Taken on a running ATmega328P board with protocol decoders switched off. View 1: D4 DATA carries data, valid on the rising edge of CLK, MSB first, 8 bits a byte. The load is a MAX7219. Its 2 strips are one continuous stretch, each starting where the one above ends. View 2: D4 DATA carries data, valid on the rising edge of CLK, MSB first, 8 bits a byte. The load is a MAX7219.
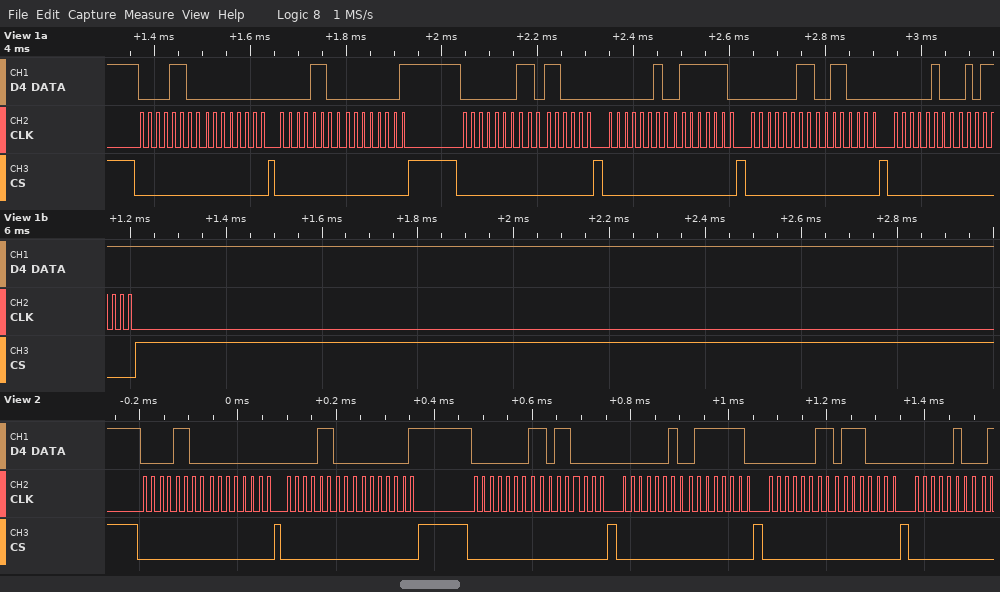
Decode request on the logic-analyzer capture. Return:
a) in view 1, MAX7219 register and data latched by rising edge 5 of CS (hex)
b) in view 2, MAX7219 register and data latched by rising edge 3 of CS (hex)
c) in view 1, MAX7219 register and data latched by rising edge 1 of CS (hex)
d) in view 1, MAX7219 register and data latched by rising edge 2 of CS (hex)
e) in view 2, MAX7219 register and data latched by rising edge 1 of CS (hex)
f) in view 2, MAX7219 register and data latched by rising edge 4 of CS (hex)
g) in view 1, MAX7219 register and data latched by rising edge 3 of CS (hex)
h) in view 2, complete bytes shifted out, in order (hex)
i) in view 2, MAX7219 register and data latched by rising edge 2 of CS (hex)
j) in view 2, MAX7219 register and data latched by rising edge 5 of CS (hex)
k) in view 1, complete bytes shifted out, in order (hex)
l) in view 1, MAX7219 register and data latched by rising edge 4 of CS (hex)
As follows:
register 0x3, data 0x30
register 0x1, data 0xB0
register 0xC, data 0x00
register 0xC, data 0x01
register 0xC, data 0x00
register 0x2, data 0x7E
register 0x1, data 0xB0
0C 00 0C 01 01 B0 02 7E 03 70 04
register 0xC, data 0x01
register 0x3, data 0x70
0C 00 0C 01 01 B0 02 7E 03 30 04 5F
register 0x2, data 0x7E
